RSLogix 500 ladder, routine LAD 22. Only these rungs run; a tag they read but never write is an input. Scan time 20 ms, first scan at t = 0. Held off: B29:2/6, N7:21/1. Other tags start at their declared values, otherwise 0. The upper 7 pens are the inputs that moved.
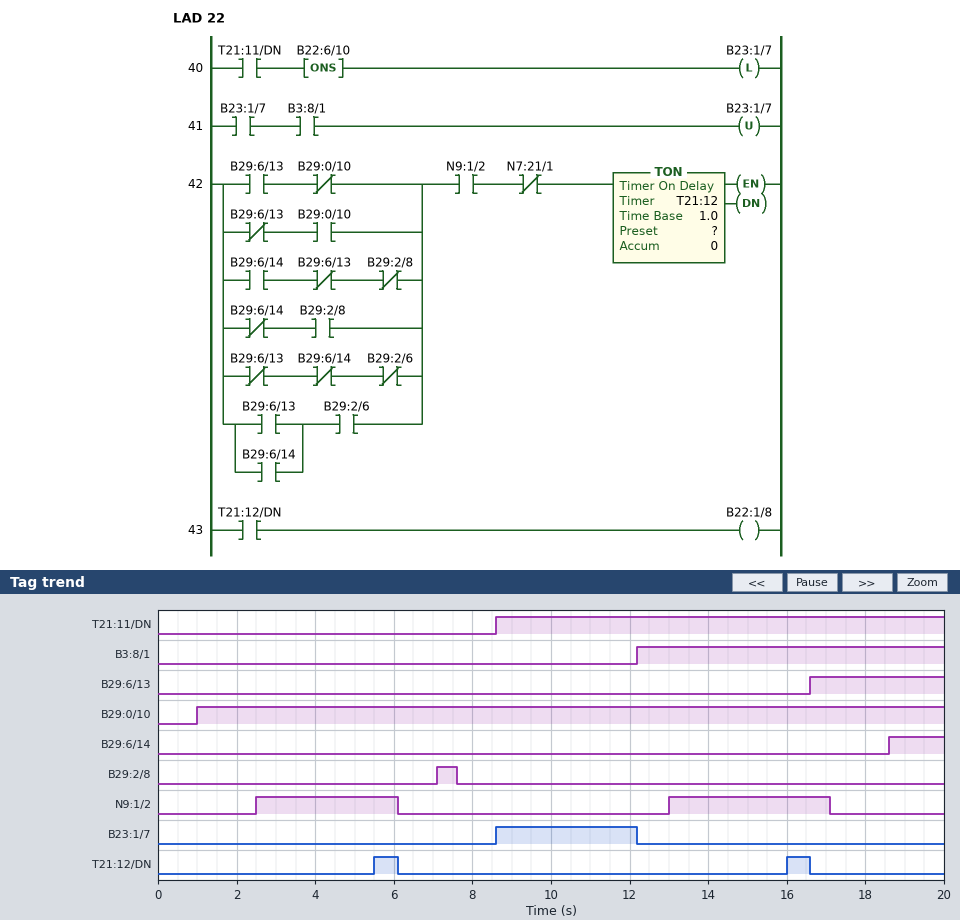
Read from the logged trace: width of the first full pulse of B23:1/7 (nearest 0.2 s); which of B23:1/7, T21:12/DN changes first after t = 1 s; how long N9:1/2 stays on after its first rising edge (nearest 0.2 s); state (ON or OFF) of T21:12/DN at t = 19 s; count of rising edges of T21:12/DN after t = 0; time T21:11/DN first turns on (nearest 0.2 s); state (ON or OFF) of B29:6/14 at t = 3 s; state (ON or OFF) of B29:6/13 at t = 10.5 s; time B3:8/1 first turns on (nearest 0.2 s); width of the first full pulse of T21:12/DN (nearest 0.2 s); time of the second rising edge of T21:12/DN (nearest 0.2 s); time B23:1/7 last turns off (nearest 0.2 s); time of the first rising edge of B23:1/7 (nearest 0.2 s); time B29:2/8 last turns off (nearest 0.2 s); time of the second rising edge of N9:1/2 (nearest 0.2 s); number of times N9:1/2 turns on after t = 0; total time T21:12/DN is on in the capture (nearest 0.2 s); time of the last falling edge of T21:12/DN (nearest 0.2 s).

3.6 s
T21:12/DN
3.6 s
OFF
2
8.6 s
OFF
OFF
12.2 s
0.6 s
16.0 s
12.2 s
8.6 s
7.6 s
13.0 s
2
1.2 s
16.6 s
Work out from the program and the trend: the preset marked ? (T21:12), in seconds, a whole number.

3 s
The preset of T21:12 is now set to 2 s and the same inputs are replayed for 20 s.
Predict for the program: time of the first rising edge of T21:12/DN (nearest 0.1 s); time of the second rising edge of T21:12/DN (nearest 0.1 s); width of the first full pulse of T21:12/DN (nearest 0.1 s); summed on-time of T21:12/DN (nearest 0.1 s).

4.5 s
15.0 s
1.6 s
3.2 s
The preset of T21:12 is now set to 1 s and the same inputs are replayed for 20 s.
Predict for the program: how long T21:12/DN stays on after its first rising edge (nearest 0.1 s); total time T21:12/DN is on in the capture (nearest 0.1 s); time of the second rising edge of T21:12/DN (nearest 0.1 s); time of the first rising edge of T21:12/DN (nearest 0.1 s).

2.6 s
5.2 s
14.0 s
3.5 s
